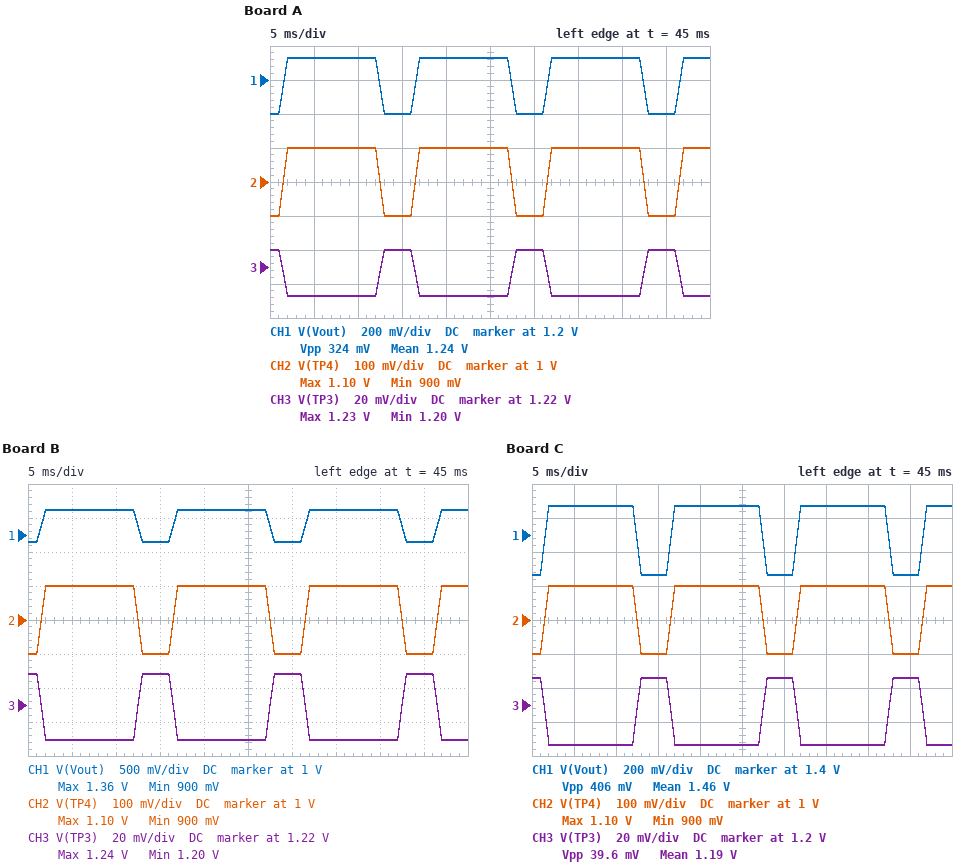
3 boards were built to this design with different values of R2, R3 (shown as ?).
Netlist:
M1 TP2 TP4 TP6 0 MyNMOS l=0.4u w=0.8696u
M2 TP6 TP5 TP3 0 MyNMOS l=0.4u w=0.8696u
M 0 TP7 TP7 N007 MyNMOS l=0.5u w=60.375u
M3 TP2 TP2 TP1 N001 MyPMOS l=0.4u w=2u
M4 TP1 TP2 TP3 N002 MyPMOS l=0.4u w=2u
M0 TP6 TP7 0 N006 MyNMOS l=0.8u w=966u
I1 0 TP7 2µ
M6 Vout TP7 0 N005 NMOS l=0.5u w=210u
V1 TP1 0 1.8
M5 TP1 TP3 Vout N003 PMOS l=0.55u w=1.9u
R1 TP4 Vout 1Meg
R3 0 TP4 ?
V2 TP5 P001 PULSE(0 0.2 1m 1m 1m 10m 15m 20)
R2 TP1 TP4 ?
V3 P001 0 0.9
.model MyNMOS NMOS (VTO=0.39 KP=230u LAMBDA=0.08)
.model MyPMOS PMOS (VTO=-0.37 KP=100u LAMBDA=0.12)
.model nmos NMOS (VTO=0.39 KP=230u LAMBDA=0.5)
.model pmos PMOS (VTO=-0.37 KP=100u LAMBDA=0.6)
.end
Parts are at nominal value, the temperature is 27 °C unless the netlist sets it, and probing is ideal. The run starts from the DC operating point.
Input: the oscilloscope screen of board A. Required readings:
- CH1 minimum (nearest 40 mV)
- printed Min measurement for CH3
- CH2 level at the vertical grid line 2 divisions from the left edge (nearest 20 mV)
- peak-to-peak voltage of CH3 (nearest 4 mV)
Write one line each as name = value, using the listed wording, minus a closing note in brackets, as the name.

CH1 minimum = 1.00 V
printed Min measurement for CH3 = 1.20 V
CH2 level at the vertical grid line 2 divisions from the left edge = 1.10 V
peak-to-peak voltage of CH3 = 28 mV
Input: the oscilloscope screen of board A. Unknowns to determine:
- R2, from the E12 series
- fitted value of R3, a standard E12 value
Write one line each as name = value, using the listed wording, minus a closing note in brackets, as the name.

R2, from the E12 series = 3.9 MΩ
fitted value of R3, a standard E12 value = 2.7 MΩ
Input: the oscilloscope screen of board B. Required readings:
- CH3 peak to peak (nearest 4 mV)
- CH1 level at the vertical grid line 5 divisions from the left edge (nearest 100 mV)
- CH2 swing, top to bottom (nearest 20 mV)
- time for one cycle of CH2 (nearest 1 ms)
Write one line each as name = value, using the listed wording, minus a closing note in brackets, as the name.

CH3 peak to peak = 40 mV
CH1 level at the vertical grid line 5 divisions from the left edge = 1.4 V
CH2 swing, top to bottom = 200 mV
time for one cycle of CH2 = 15 ms
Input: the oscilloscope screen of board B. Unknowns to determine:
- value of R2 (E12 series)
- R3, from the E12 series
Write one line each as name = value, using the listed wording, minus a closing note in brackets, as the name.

value of R2 = 1.5 MΩ
R3, from the E12 series = 1.5 MΩ
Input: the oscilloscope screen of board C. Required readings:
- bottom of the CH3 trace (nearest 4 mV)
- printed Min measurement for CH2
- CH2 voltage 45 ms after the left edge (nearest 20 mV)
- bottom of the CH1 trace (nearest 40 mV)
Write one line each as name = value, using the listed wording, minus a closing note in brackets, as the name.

bottom of the CH3 trace = 1.176 V
printed Min measurement for CH2 = 900 mV
CH2 voltage 45 ms after the left edge = 900 mV
bottom of the CH1 trace = 1.16 V
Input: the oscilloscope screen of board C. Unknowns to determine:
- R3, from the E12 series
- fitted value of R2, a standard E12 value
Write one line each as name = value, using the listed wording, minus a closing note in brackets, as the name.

R3, from the E12 series = 1.5 MΩ
fitted value of R2, a standard E12 value = 2.7 MΩ
